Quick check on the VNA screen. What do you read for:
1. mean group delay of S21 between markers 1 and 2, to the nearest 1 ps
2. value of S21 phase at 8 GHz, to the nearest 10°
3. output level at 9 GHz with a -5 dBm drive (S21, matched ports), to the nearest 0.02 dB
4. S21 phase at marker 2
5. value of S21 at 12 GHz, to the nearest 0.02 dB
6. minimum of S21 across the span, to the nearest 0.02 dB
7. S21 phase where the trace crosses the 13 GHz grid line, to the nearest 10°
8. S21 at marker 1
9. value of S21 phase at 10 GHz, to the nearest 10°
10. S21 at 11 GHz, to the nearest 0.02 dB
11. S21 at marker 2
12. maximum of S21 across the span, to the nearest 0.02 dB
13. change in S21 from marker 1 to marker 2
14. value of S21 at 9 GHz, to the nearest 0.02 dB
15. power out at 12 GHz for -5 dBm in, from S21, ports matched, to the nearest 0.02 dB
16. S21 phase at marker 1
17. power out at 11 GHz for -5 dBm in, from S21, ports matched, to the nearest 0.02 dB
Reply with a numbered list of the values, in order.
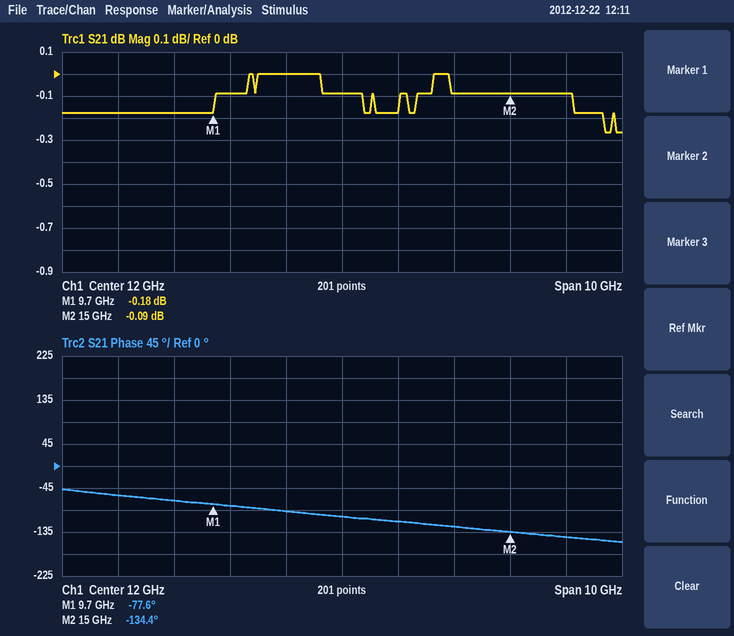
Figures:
1. 30 ps
2. -60°
3. -5.18 dBm
4. -134.4°
5. -0.08 dB
6. -0.26 dB
7. -110°
8. -0.18 dB
9. -80°
10. 0.00 dB
11. -0.09 dB
12. 0.00 dB
13. 0.09 dB
14. -0.18 dB
15. -5.08 dBm
16. -77.6°
17. -5.00 dBm
